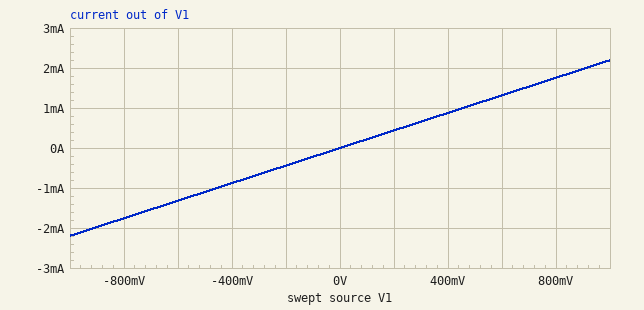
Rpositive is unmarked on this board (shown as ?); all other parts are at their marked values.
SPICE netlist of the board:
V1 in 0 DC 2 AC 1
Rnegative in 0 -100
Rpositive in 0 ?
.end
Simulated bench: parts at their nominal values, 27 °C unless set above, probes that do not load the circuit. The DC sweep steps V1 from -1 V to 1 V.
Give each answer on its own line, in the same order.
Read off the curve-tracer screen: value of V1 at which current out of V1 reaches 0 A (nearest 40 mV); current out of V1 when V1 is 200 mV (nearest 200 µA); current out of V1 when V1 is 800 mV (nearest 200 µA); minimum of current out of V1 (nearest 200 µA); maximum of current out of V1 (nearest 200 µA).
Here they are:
0 V
400 µA
1.8 mA
-2.2 mA
2.2 mA
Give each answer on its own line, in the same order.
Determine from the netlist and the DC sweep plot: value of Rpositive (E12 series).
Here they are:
82 Ω
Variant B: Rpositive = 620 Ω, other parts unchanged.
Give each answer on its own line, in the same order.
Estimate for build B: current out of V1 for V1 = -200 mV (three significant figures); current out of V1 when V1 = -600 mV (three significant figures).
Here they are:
1.68 mA
5.03 mA
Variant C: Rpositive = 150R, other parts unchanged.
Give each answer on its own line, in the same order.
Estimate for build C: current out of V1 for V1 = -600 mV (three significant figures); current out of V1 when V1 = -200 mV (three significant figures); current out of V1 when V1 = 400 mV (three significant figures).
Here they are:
2.00 mA
667 µA
-1.33 mA
